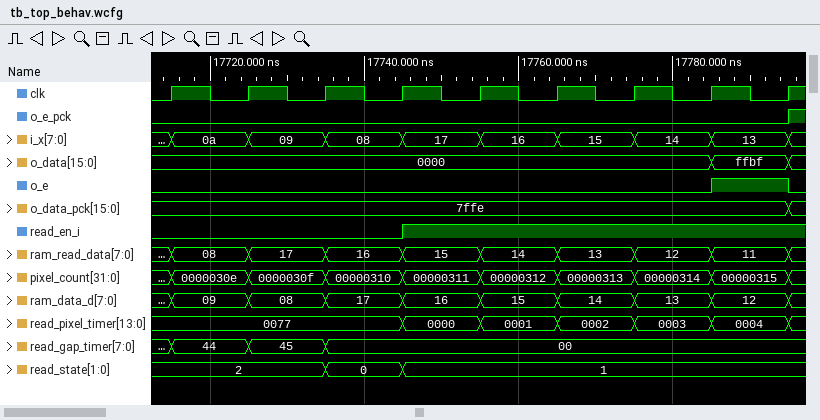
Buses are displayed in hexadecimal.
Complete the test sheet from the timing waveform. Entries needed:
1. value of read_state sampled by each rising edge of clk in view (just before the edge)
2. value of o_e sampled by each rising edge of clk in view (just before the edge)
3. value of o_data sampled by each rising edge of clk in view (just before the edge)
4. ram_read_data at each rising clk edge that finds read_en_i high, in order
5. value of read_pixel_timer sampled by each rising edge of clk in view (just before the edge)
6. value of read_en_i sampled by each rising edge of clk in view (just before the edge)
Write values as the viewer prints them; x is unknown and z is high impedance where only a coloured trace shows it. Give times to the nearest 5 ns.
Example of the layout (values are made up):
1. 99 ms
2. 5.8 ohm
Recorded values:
1. 2, 2, 2, 0, 1, 1, 1, 1, 1
2. 0 0 0 0 0 0 0 0 1
3. 0000, 0000, 0000, 0000, 0000, 0000, 0000, 0000, ffbf
4. 15, 14, 13, 12, 11
5. 0077, 0077, 0077, 0077, 0000, 0001, 0002, 0003, 0004
6. 0 0 0 0 1 1 1 1 1
